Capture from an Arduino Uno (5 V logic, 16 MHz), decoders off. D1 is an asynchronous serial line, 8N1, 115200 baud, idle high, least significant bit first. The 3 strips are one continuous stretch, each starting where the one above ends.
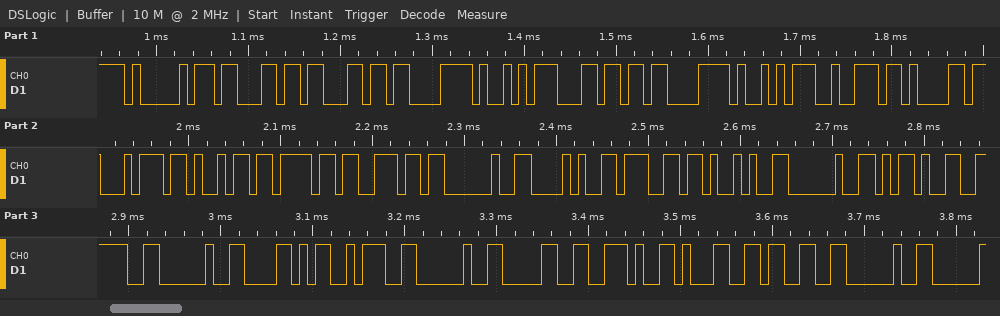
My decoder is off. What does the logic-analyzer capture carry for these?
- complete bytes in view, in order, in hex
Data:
41 63 63 C3 A9 6C C3 A9 72 61 74 69 6F 6E 20 28 67 29 20 2D 3E 20 58 3A 20 30 2E 31 33 20
